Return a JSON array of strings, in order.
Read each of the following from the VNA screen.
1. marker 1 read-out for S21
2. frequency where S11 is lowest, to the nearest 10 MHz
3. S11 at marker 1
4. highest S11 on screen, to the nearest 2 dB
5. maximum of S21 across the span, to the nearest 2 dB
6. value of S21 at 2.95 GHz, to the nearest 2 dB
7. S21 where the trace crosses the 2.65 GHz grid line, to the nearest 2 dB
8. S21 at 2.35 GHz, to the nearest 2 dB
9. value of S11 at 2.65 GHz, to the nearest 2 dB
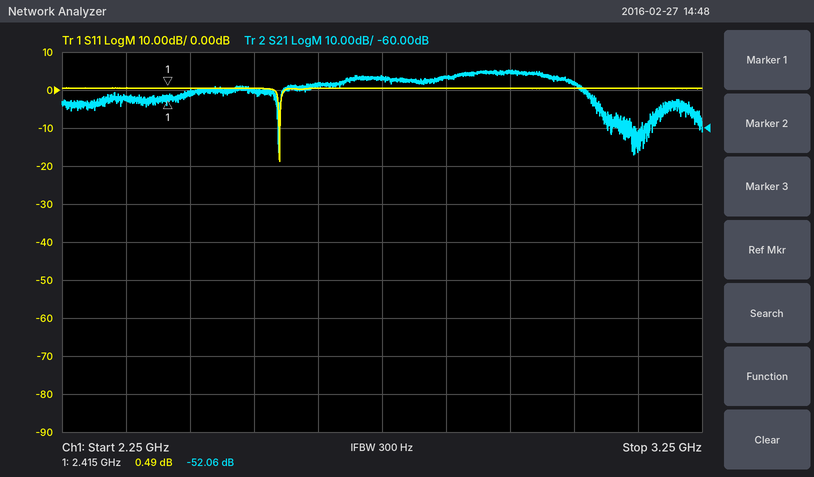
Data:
["-52.06 dB", "2.59 GHz", "0.49 dB", "0 dB", "-44 dB", "-46 dB", "-48 dB", "-52 dB", "0 dB"]
